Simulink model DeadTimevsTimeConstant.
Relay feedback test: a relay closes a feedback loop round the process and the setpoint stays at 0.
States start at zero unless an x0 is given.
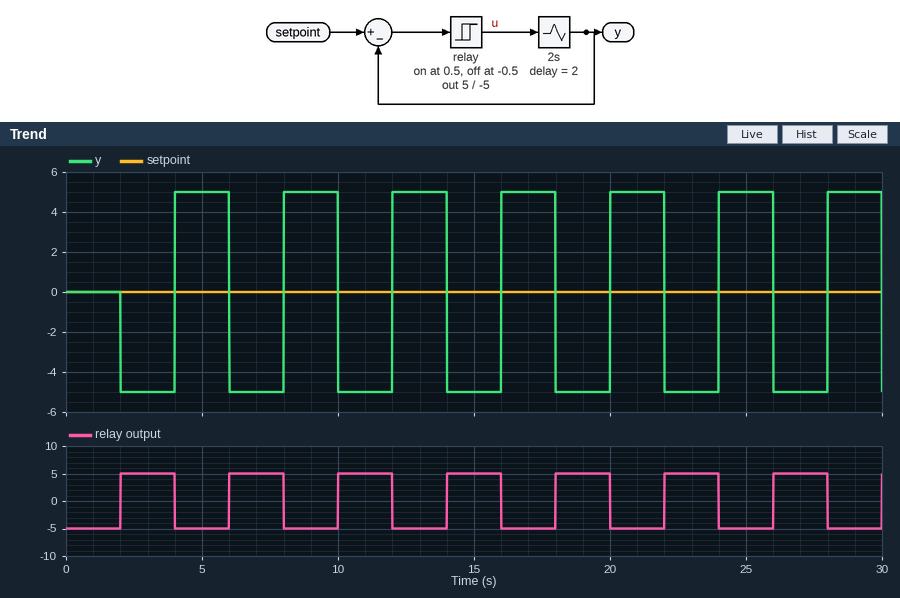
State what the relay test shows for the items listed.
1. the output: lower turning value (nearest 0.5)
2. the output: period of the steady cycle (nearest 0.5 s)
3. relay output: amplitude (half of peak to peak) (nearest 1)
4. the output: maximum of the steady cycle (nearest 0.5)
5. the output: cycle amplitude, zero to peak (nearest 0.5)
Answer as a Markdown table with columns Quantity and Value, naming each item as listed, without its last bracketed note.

| Quantity | Value |
|---|---|
| the output: lower turning value | -5.0 |
| the output: period of the steady cycle | 4.0 s |
| relay output: amplitude (half of peak to peak) | 5 |
| the output: maximum of the steady cycle | 5.0 |
| the output: cycle amplitude, zero to peak | 5.0 |
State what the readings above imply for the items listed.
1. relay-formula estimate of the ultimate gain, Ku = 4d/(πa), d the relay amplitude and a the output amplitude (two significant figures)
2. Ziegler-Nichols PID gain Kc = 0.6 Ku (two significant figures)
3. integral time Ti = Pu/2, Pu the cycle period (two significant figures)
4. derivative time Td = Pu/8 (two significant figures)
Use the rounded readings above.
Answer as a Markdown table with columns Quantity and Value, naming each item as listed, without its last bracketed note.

| Quantity | Value |
|---|---|
| relay-formula estimate of the ultimate gain, Ku = 4d/(πa), d the relay amplitude and a the output amplitude | 1.3 |
| Ziegler-Nichols PID gain Kc = 0.6 Ku | 0.78 |
| integral time Ti = Pu/2, Pu the cycle period | 2.0 s |
| derivative time Td = Pu/8 | 0.50 s |
